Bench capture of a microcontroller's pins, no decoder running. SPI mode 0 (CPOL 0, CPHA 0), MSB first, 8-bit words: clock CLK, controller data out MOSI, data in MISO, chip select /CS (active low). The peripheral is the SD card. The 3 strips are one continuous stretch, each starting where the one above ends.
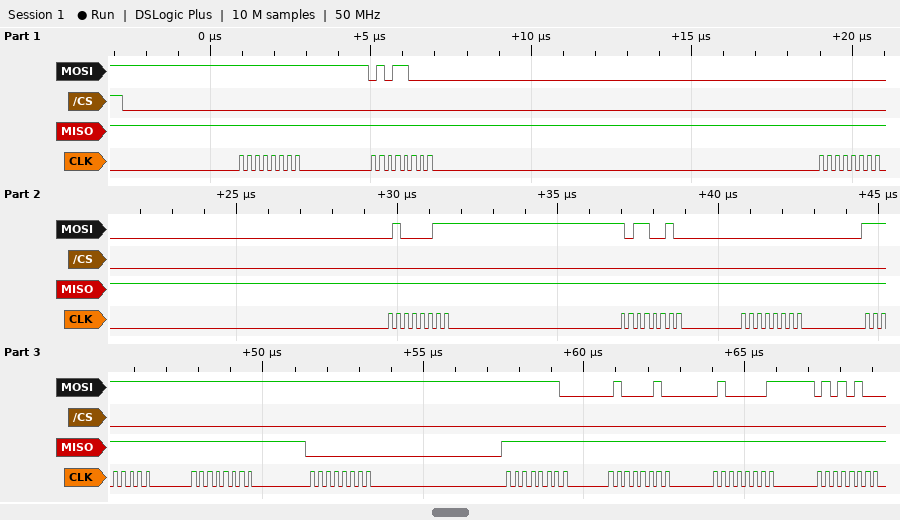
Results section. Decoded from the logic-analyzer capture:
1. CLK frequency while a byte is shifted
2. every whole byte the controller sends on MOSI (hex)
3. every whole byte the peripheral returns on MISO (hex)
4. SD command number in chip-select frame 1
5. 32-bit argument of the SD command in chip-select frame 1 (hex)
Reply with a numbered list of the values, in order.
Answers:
1. 4 MHz
2. FF 58 00 43 B2 00 FF FF FF FE 42 41 54
3. FF FF FF FF FF FF FF FF 00 FF FF FF FF
4. CMD24
5. 0x0043B200
